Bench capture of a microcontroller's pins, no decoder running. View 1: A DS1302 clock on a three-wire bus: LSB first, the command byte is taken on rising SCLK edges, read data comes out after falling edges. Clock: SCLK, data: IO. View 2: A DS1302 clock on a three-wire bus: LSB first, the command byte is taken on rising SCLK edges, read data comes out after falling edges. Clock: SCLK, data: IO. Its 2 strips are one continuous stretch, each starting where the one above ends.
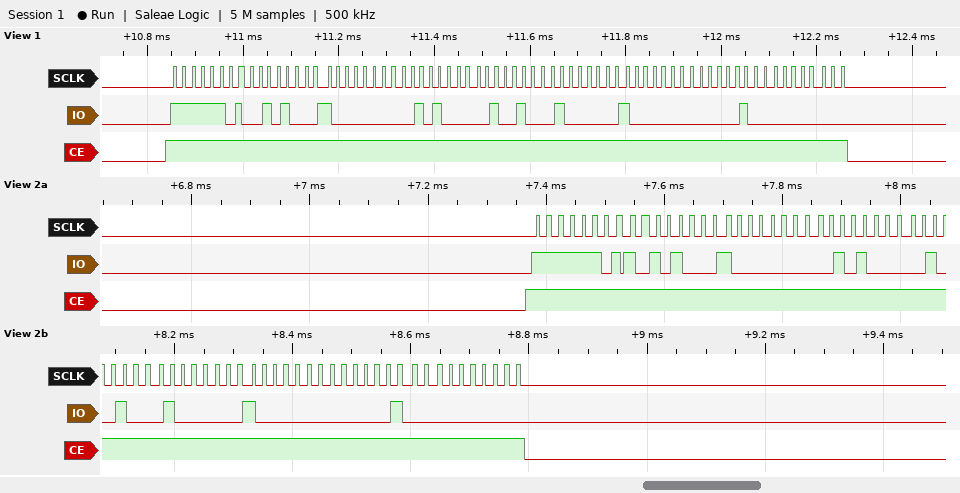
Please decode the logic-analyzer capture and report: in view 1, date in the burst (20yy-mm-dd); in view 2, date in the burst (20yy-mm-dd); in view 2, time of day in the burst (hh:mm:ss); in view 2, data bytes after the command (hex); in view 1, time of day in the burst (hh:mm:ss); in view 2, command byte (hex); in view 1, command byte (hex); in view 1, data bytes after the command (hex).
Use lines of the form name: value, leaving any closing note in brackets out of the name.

in view 1, date in the burst: 2020-02-24
in view 2, date in the burst: 2020-02-24
in view 2, time of day in the burst: 14:01:15
in view 2, data bytes after the command: 15 01 14 24 02 01 20 00
in view 1, time of day in the burst: 14:01:14
in view 2, command byte: 0xBF
in view 1, command byte: 0xBF
in view 1, data bytes after the command: 14 01 14 24 02 01 20 00
